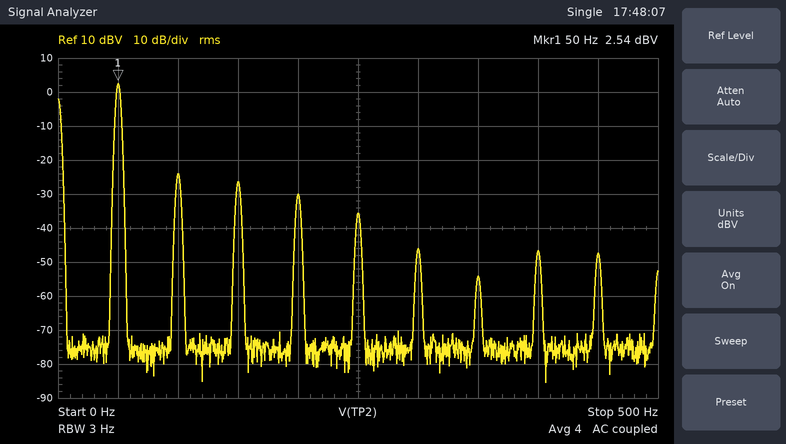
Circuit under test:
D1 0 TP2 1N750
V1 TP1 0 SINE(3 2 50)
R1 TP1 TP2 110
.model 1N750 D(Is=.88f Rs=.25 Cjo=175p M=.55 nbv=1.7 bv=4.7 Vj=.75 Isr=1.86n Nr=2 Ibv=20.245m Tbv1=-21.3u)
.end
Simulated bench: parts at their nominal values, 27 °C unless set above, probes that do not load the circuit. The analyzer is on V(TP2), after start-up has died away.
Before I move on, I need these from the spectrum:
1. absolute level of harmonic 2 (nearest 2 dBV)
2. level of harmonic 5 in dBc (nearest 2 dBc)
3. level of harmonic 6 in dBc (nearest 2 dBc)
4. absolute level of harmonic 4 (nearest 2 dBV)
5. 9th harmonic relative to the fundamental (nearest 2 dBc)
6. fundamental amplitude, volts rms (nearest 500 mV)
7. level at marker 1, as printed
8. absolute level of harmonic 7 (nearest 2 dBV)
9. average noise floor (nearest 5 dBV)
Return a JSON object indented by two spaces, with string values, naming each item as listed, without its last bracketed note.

{
  "absolute level of harmonic 2": "-24 dBV",
  "level of harmonic 5 in dBc": "-38 dBc",
  "level of harmonic 6 in dBc": "-48 dBc",
  "absolute level of harmonic 4": "-30 dBV",
  "9th harmonic relative to the fundamental": "-50 dBc",
  "fundamental amplitude, volts rms": "1.5 V",
  "level at marker 1, as printed": "2.54 dBV",
  "absolute level of harmonic 7": "-54 dBV",
  "average noise floor": "-75 dBV"
}
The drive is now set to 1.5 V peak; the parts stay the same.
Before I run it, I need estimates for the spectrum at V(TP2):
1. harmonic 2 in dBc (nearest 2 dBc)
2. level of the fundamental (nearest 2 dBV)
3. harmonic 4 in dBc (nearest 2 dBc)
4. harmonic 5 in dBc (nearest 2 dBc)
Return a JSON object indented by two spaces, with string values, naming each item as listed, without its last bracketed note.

{
  "harmonic 2 in dBc": "-56 dBc",
  "level of the fundamental": "0 dBV",
  "harmonic 4 in dBc": "-58 dBc",
  "harmonic 5 in dBc": "-60 dBc"
}
